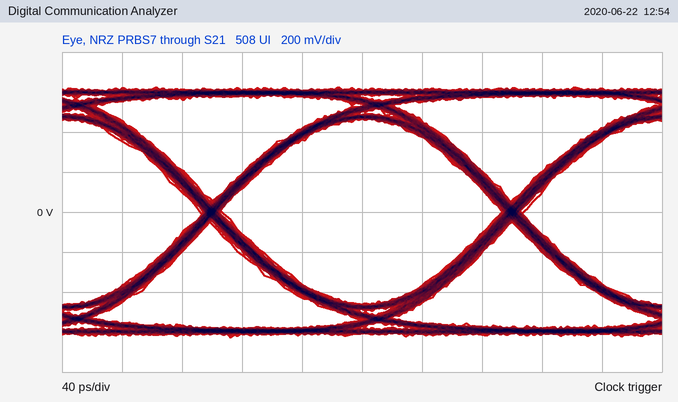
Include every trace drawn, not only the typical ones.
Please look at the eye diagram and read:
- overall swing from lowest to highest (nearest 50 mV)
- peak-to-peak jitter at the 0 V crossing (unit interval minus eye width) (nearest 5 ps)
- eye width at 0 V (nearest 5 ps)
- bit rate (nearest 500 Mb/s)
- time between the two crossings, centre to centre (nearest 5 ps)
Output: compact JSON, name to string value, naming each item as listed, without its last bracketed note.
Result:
{"overall swing from lowest to highest": "1.25 V", "peak-to-peak jitter at the 0 V crossing (unit interval minus eye width)": "15 ps", "eye width at 0 V": "185 ps", "bit rate": "5.0 Gb/s", "time between the two crossings, centre to centre": "200 ps"}
